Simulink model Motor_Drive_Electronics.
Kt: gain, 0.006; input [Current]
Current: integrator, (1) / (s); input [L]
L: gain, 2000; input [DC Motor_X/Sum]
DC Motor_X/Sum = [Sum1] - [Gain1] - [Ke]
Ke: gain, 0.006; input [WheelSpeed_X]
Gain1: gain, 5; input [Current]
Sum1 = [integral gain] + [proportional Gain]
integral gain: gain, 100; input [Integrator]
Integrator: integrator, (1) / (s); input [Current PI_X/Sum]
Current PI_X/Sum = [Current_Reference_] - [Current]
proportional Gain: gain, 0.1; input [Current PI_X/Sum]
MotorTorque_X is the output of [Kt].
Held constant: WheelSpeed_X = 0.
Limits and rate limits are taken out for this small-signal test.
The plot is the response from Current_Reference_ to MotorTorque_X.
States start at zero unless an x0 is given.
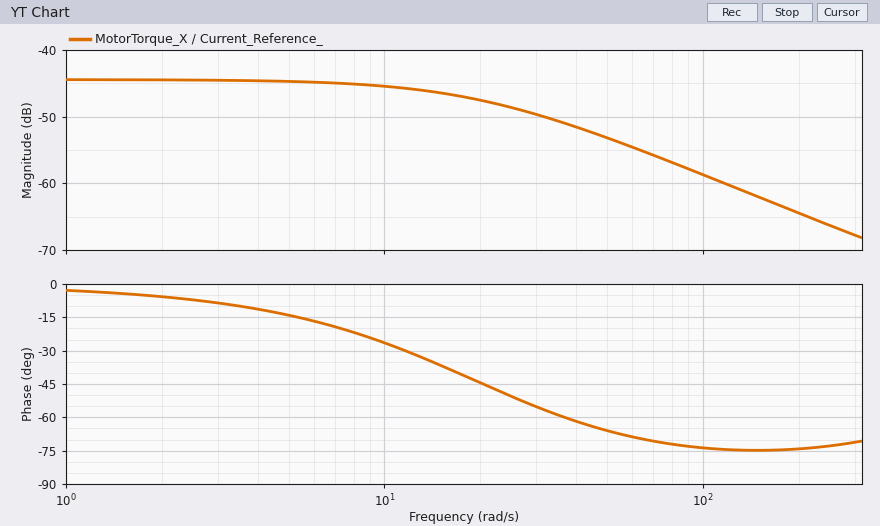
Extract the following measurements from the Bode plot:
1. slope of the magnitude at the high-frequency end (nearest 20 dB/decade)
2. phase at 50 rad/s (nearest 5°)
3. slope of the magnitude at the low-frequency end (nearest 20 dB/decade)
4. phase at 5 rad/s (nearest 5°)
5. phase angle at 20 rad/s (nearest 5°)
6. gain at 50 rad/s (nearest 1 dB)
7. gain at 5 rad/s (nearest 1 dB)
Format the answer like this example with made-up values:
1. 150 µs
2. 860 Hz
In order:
1. -20 dB/decade
2. -65°
3. 0 dB/decade
4. -15°
5. -45°
6. -53 dB
7. -45 dB
